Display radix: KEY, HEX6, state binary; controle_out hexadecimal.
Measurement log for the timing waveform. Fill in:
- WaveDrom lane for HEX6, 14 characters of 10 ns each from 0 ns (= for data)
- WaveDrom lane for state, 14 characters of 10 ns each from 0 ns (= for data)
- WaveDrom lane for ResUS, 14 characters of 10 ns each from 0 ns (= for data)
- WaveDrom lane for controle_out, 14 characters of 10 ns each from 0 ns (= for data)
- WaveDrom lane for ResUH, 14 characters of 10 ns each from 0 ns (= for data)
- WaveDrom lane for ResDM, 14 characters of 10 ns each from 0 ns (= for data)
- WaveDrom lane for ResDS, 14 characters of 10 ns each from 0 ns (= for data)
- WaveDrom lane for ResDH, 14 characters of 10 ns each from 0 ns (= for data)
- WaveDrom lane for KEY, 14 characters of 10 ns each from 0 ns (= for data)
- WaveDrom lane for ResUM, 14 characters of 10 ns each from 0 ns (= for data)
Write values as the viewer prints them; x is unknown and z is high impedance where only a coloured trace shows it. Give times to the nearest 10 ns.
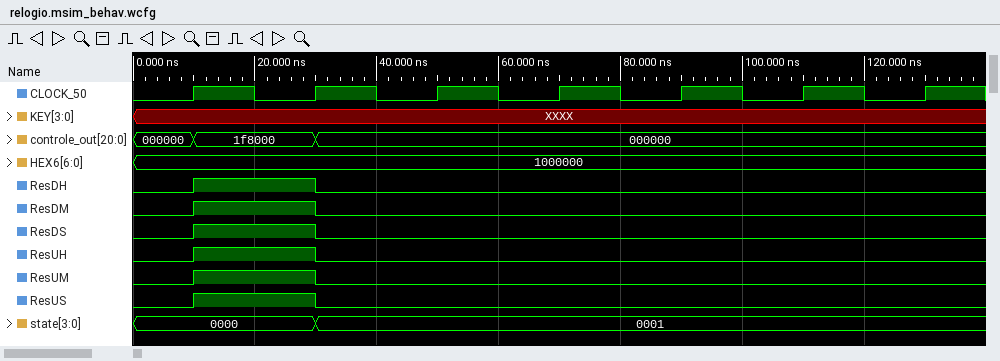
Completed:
{name: 'HEX6', wave: '=.............', data: '1000000'}
{name: 'state', wave: '=..=..........', data: '0000 0001'}
{name: 'ResUS', wave: '01.0..........'}
{name: 'controle_out', wave: '==.=..........', data: '000000 1f8000 000000'}
{name: 'ResUH', wave: '01.0..........'}
{name: 'ResDM', wave: '01.0..........'}
{name: 'ResDS', wave: '01.0..........'}
{name: 'ResDH', wave: '01.0..........'}
{name: 'KEY', wave: 'x.............'}
{name: 'ResUM', wave: '01.0..........'}
